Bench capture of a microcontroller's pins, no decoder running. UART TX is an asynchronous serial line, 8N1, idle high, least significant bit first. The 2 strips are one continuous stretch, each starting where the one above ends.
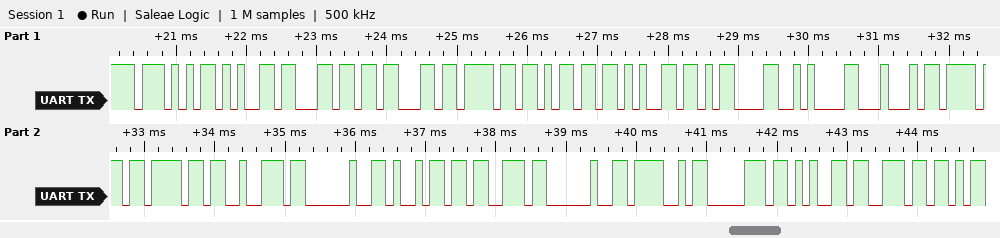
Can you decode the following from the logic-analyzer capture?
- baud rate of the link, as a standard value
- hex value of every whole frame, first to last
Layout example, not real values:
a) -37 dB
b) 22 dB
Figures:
a) 9600 baud
b) 57 65 6C 63 6F 6D 65 0D 0A 44 6F 6F 72 20 69 73 20 4F 70 65 6E
